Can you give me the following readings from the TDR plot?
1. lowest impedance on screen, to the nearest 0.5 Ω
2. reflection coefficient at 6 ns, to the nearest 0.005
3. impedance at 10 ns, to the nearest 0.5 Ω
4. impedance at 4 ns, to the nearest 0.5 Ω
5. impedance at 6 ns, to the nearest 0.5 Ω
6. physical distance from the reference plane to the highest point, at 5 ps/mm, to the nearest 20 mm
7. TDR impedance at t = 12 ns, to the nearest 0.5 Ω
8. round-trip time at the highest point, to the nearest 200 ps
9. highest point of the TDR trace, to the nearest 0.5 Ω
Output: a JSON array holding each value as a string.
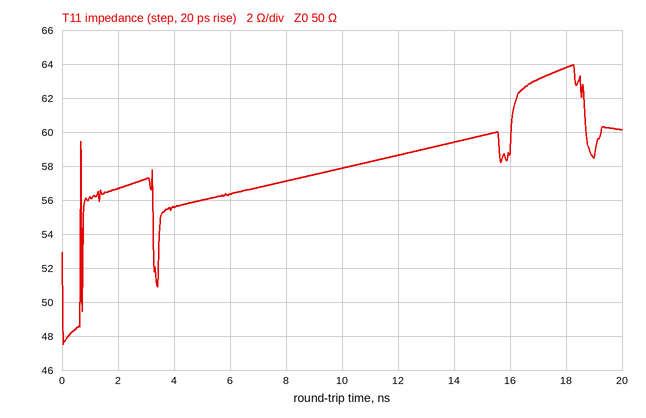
["47.5 Ω", "+0.060", "58.0 Ω", "55.5 Ω", "56.5 Ω", "1.82 m", "58.5 Ω", "18.2 ns", "64.0 Ω"]
